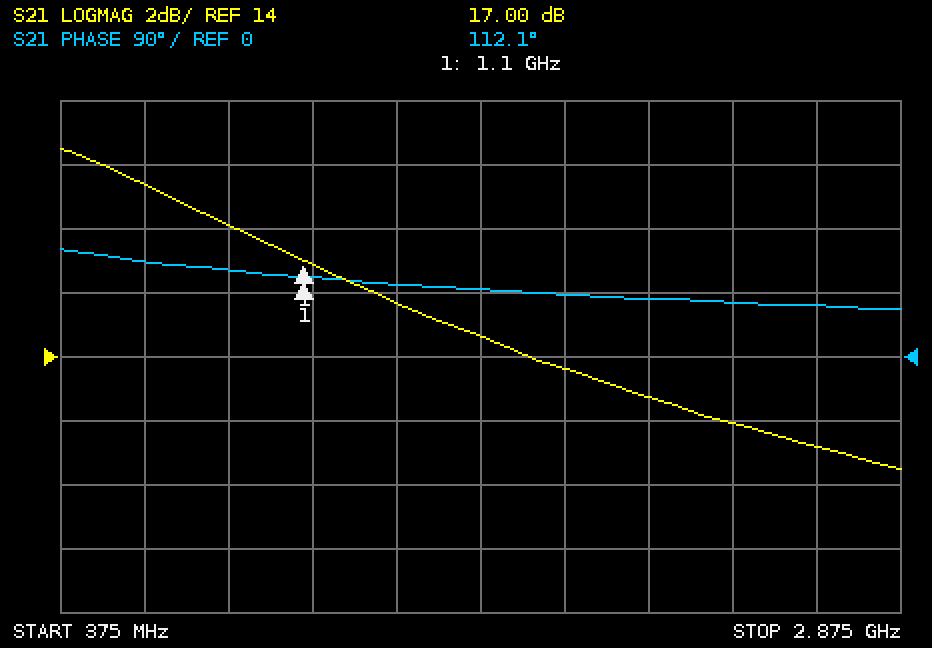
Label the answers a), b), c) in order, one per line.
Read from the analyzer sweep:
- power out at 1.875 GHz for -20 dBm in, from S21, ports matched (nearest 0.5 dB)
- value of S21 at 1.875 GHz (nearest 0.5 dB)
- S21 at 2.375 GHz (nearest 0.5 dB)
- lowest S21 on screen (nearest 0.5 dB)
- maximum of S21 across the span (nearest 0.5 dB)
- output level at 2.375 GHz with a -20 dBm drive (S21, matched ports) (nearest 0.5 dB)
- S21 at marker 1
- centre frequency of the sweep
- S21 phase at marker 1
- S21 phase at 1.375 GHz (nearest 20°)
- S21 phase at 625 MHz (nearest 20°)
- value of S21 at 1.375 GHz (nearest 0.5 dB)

a) -6.5 dBm
b) 13.5 dB
c) 12.0 dB
d) 10.5 dB
e) 20.5 dB
f) -8.0 dBm
g) 17.00 dB
h) 1.625 GHz
i) 112.1°
j) 100°
k) 140°
l) 15.5 dB
